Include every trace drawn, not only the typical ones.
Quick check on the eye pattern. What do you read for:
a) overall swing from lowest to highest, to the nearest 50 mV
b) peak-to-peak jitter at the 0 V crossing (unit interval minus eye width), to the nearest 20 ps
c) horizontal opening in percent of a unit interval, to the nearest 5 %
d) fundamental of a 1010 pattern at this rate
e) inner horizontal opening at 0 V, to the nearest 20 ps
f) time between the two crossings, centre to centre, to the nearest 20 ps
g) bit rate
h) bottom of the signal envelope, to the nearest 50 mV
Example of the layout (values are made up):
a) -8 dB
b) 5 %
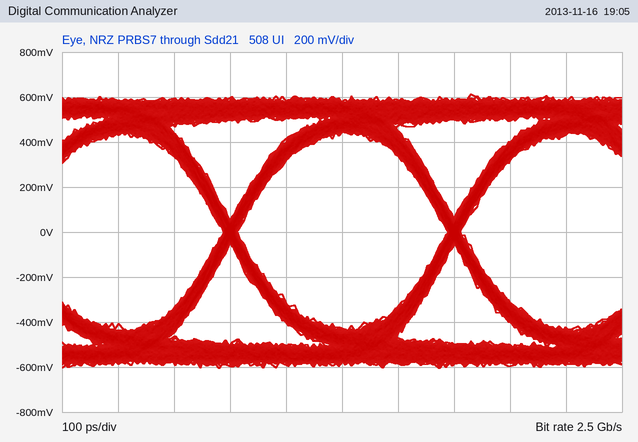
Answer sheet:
a) 1.20 V
b) 20 ps
c) 95 %
d) 1.25 GHz
e) 380 ps
f) 400 ps
g) 2.5 Gb/s
h) -600 mV
